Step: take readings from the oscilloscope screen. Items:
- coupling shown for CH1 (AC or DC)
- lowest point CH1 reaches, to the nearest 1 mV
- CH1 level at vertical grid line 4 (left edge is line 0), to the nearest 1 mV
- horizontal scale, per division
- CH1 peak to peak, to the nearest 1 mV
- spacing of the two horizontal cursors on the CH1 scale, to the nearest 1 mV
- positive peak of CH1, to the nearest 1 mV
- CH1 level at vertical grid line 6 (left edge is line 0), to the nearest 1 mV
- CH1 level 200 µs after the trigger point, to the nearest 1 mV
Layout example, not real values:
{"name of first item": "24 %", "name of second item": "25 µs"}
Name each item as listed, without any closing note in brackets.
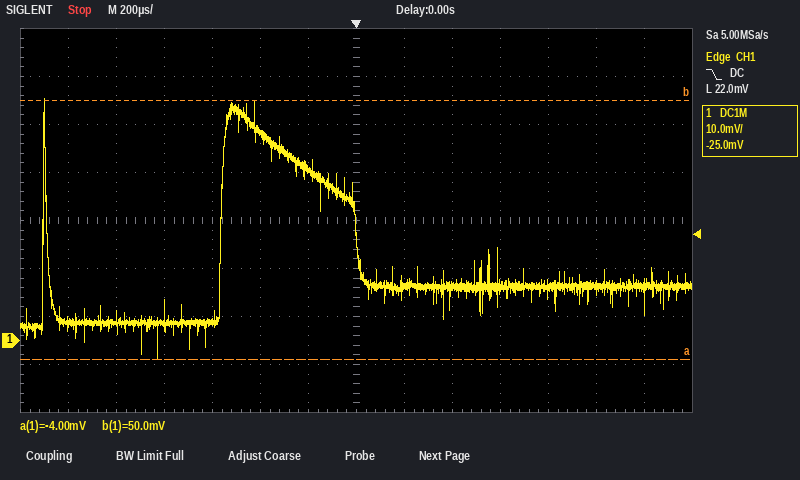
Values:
{"coupling shown for CH1": "DC", "lowest point CH1 reaches, to the nearest 1 mV": "-4 mV", "CH1 level at vertical grid line 4 (left edge is line 0), to the nearest 1 mV": "4 mV", "horizontal scale, per division": "200 µs", "CH1 peak to peak, to the nearest 1 mV": "54 mV", "spacing of the two horizontal cursors on the CH1 scale, to the nearest 1 mV": "54 mV", "positive peak of CH1, to the nearest 1 mV": "50 mV", "CH1 level at vertical grid line 6 (left edge is line 0), to the nearest 1 mV": "36 mV", "CH1 level 200 µs after the trigger point, to the nearest 1 mV": "11 mV"}
